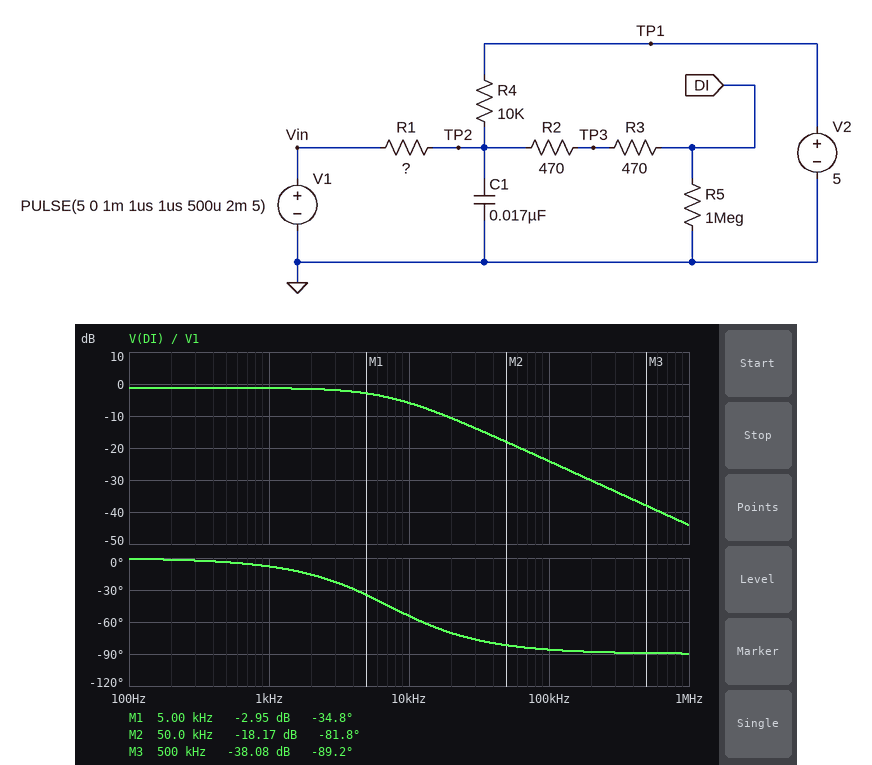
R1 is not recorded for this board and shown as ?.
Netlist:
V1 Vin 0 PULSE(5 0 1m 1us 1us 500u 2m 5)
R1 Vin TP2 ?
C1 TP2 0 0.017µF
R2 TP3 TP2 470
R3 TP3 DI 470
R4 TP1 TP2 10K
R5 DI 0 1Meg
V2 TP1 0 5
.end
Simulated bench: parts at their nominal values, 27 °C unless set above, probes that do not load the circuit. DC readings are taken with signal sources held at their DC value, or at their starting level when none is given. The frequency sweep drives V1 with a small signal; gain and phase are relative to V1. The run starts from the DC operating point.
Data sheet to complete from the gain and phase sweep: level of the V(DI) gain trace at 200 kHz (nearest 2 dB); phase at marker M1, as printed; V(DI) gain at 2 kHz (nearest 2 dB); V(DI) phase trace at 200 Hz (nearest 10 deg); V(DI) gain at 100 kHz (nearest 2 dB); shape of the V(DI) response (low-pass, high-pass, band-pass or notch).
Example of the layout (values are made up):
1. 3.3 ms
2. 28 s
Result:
1. -30 dB
2. -34.8 deg
3. -2 dB
4. 0 deg
5. -24 dB
6. low-pass
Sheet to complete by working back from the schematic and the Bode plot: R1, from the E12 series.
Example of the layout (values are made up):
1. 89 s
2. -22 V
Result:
1. 1.5 kΩ
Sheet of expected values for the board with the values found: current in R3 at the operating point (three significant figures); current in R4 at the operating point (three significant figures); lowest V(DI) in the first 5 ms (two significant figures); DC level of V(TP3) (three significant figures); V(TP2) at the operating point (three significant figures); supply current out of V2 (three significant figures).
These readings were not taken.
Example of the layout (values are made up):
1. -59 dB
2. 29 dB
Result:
1. 4.99 µA
2. 651 nA
3. 650 mV
4. 4.99 V
5. 4.99 V
6. 651 nA
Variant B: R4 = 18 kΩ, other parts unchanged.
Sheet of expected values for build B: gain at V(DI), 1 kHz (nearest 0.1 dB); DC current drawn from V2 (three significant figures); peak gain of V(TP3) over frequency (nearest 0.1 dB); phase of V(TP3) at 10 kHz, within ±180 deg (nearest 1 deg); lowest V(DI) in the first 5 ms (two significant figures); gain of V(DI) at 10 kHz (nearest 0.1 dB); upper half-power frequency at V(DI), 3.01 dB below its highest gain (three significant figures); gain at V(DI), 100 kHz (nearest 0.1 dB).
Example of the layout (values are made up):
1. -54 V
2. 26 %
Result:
1. -0.8 dB
2. 384 nA
3. -0.7 dB
4. -56 deg
5. 380 mV
6. -5.7 dB
7. 6.77 kHz
8. -24.1 dB
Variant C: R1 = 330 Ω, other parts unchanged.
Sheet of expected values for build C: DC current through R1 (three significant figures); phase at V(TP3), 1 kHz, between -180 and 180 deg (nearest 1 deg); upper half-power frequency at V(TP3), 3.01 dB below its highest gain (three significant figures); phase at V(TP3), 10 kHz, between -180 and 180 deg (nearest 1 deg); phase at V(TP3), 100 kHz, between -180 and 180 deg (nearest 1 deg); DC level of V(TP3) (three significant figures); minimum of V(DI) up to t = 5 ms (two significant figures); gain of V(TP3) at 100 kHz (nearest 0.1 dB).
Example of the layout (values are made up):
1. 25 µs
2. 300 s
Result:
1. 4.83 µA
2. -2 deg
3. 29.3 kHz
4. -19 deg
5. -74 deg
6. 5.00 V
7. 160 mV
8. -11.3 dB
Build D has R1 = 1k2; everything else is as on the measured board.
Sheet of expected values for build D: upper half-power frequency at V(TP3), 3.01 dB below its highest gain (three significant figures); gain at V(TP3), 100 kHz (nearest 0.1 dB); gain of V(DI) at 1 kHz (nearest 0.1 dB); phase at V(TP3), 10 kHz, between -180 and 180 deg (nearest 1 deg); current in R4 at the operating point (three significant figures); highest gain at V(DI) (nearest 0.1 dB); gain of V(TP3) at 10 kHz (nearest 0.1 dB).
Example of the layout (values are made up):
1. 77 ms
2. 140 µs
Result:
1. 8.75 kHz
2. -22.2 dB
3. -1.1 dB
4. -49 deg
5. 535 nA
6. -1.0 dB
7. -4.6 dB
